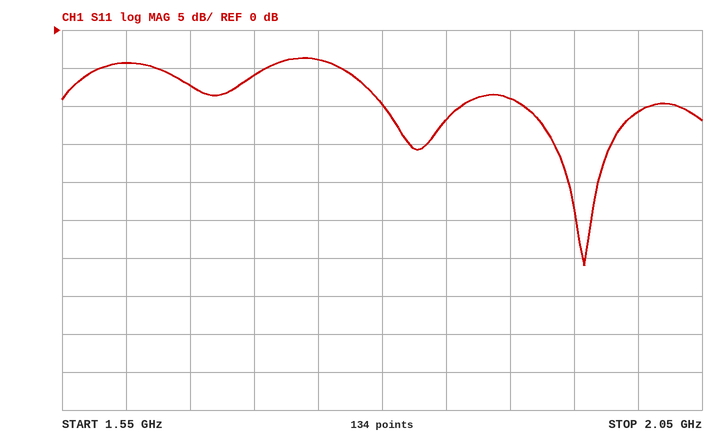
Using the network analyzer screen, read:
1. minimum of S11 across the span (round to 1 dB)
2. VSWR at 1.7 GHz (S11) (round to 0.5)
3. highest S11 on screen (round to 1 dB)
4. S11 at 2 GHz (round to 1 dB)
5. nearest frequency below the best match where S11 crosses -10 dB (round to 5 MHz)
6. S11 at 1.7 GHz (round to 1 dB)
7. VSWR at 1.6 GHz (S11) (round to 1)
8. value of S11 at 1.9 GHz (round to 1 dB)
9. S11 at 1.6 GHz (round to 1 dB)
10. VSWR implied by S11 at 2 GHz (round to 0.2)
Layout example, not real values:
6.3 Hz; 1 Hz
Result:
-31 dB; 3.0; -4 dB; -11 dB; 1.910 GHz; -6 dB; 4; -9 dB; -4 dB; 1.8
